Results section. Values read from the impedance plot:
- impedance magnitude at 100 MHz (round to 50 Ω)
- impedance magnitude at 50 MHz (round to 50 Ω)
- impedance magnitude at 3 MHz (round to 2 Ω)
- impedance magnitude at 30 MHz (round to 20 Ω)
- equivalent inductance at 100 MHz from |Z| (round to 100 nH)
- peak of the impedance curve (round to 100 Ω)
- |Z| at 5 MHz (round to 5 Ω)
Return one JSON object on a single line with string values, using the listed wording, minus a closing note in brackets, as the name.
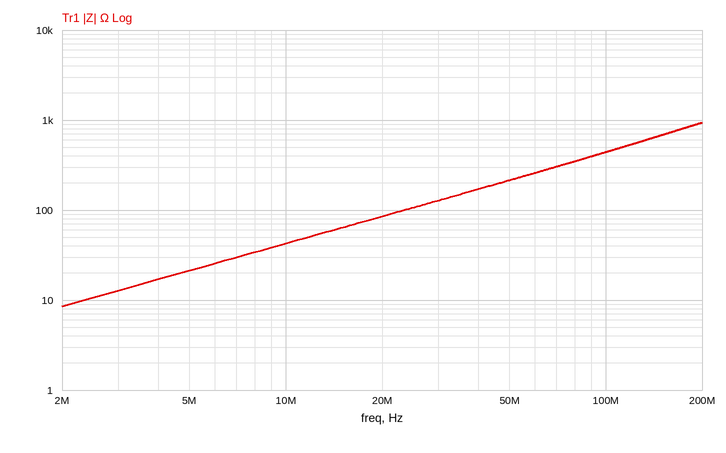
{"impedance magnitude at 100 MHz": "450 Ω", "impedance magnitude at 50 MHz": "200 Ω", "impedance magnitude at 3 MHz": "12 Ω", "impedance magnitude at 30 MHz": "120 Ω", "equivalent inductance at 100 MHz from |Z|": "700 nH", "peak of the impedance curve": "900 Ω", "|Z| at 5 MHz": "20 Ω"}
